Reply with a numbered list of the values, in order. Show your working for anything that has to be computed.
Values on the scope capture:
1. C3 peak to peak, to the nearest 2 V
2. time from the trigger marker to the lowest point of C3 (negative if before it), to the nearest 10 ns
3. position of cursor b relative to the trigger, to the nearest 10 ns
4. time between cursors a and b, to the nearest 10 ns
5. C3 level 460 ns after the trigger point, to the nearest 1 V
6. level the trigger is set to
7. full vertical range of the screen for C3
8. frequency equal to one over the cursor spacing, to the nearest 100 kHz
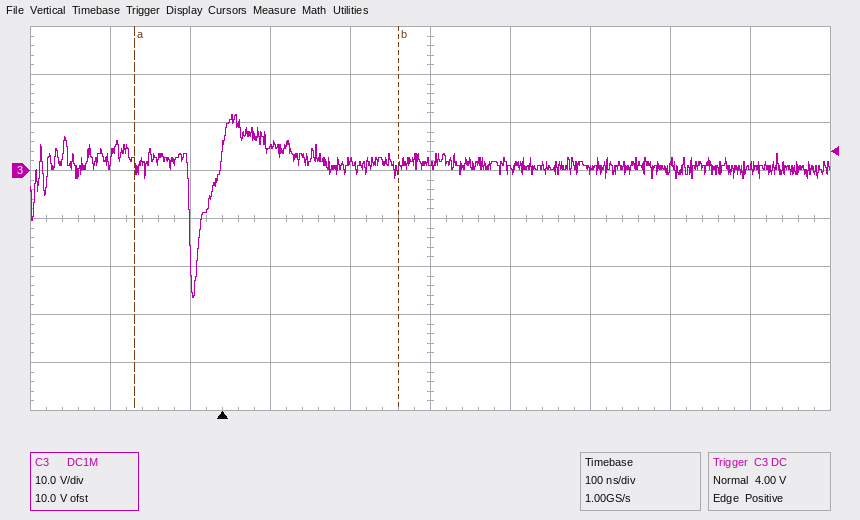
1. 38 V
2. -40 ns
3. +220 ns
4. 330 ns
5. 0 V
6. 4.00 V
7. 80 V
8. 1 / 330 ns ≈ 3.0 MHz
